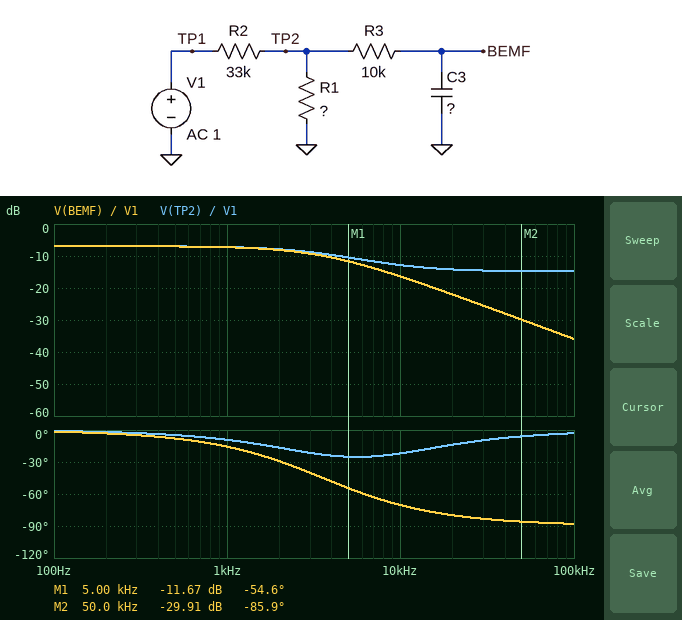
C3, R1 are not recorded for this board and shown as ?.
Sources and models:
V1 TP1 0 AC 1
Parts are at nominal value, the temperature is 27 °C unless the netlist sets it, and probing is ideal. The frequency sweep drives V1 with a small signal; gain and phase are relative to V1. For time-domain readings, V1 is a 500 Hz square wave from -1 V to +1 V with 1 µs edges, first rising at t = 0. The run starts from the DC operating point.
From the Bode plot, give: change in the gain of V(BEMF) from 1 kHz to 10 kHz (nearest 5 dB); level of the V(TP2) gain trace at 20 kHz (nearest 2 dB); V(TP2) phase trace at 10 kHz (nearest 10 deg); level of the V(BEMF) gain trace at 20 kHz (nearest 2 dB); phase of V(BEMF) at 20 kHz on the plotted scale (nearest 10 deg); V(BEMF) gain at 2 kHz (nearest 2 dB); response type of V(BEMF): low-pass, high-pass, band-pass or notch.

-10 dB
-14 dB
-20 deg
-22 dB
-80 deg
-8 dB
low-pass
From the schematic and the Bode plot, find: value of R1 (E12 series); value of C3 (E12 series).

27 kΩ
1.8 nF
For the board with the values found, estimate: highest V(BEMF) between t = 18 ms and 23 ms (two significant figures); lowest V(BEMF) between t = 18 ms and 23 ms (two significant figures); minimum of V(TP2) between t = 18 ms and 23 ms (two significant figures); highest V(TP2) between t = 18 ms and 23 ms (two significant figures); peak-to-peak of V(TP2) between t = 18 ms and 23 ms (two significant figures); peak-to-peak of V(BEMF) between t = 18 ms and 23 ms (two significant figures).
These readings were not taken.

450 mV
-450 mV
-450 mV
450 mV
900 mV
900 mV
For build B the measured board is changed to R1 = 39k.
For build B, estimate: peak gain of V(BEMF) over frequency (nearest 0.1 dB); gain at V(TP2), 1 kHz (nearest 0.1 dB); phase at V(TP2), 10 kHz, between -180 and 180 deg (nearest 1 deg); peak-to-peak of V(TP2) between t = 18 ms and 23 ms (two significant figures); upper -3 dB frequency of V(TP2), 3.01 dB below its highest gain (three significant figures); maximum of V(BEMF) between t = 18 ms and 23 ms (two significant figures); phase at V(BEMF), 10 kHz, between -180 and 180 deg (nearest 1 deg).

-5.3 dB
-5.7 dB
-24 deg
1.1 V
3.68 kHz
540 mV
-72 deg
